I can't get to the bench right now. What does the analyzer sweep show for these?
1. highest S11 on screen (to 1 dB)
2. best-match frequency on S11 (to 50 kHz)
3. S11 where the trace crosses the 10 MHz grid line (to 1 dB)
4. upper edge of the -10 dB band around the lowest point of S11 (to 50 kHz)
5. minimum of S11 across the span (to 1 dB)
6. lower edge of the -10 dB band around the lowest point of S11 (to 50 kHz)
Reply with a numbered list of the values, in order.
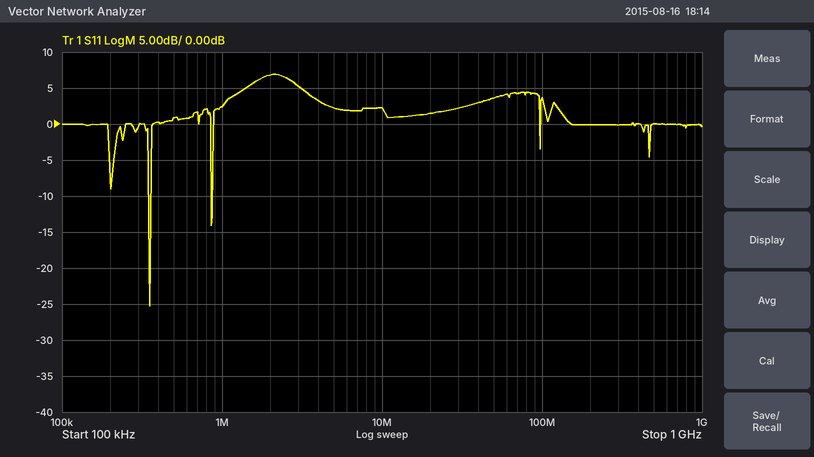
1. 7 dB
2. 350 kHz
3. 2 dB
4. 350 kHz
5. -25 dB
6. 350 kHz
